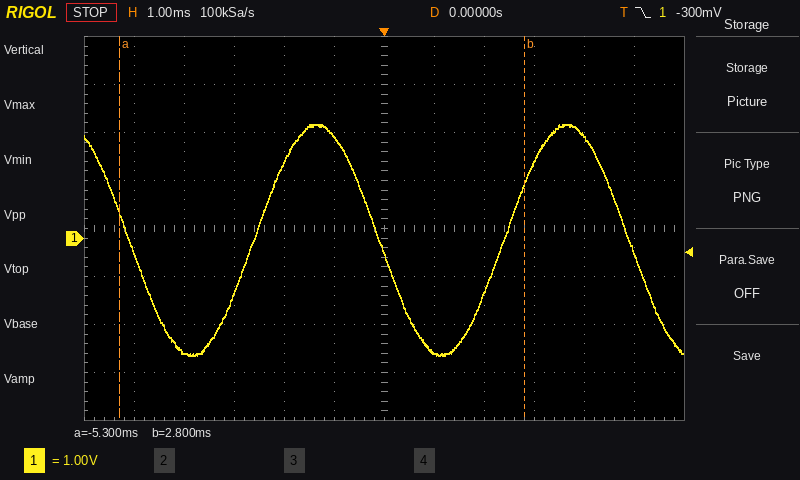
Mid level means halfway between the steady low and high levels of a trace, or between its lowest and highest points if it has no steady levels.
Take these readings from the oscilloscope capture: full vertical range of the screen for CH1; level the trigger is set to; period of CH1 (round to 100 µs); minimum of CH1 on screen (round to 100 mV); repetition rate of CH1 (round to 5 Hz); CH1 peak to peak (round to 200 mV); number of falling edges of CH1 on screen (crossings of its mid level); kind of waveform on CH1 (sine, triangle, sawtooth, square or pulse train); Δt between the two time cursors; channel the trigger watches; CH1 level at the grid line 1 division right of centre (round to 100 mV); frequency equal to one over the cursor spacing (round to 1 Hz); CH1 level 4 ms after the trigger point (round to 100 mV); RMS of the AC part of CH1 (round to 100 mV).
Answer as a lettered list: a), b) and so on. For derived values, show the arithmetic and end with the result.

a) 8 V
b) -300 mV
c) 5.0 ms
d) -2.4 V
e) 1 / 5.0 ms ≈ 200 Hz
f) 4.8 V
g) 3
h) sine
i) 2.8 ms − (-5.3 ms) = 8.1 ms
j) CH1
k) -2.4 V
l) 1 / 8.1 ms ≈ 123 Hz
m) 2.1 V
n) 4.8 V / (2√2) ≈ 1.7 V
